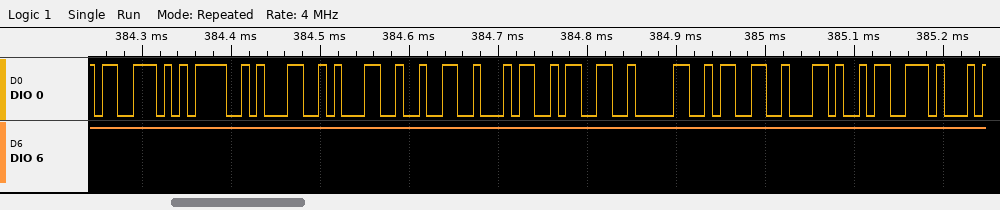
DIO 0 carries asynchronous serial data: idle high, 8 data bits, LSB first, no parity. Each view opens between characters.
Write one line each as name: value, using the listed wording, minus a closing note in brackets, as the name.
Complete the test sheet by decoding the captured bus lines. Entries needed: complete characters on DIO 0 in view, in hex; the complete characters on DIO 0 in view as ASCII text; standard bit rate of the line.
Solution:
complete characters on DIO 0 in view, in hex: 73, 3D, 31, 31, 32, 34, 33, 30, 33, 2C, 73
the complete characters on DIO 0 in view as ASCII text: "s=1124303,s"
standard bit rate of the line: 115200 baud
